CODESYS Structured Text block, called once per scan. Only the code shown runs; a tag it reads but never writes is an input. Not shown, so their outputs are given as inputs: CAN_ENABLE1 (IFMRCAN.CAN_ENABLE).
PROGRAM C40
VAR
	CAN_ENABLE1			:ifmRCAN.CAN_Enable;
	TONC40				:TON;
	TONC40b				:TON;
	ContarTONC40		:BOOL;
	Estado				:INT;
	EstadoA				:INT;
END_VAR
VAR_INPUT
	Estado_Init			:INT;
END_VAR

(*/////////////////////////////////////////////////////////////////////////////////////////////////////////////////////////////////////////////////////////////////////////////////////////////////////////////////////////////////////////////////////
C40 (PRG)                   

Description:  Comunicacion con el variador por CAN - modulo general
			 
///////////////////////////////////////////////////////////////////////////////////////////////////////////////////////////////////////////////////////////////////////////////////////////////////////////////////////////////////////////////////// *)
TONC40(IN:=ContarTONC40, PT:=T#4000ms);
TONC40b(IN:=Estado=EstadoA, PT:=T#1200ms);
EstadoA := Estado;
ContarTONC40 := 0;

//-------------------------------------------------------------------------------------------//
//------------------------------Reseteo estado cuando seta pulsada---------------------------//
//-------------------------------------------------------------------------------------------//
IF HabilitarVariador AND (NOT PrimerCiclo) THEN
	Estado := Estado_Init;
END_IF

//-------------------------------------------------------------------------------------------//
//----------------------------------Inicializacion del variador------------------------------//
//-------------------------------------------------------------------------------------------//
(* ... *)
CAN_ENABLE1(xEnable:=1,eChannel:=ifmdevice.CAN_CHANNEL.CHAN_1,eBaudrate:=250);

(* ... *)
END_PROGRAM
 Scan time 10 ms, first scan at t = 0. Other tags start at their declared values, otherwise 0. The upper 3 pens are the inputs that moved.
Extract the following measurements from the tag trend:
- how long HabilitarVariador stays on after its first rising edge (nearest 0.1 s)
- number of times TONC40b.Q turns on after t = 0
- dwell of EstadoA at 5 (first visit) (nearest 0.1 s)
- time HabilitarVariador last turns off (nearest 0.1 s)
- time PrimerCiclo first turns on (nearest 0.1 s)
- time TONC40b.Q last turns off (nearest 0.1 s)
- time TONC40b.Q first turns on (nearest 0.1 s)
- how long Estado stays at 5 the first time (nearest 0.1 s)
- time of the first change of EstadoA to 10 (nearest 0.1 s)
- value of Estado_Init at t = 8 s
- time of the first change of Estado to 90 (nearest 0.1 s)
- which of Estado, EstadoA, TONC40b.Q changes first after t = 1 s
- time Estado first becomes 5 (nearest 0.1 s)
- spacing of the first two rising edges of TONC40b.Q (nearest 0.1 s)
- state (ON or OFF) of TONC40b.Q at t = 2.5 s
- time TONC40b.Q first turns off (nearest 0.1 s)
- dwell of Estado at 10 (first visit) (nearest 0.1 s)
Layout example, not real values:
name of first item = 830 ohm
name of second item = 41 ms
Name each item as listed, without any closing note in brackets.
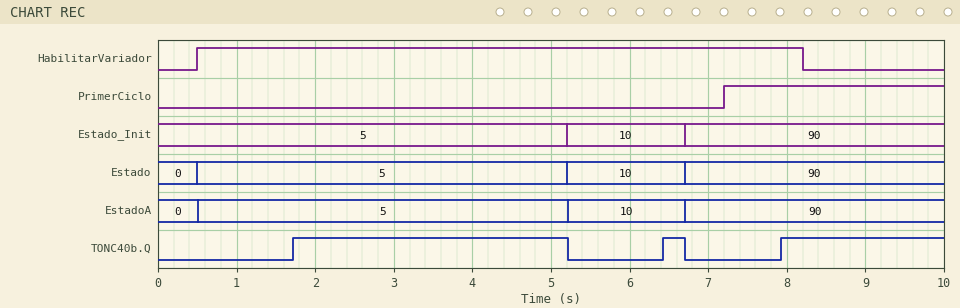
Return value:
how long HabilitarVariador stays on after its first rising edge = 7.7 s
number of times TONC40b.Q turns on after t = 0 = 3
dwell of EstadoA at 5 (first visit) = 4.7 s
time HabilitarVariador last turns off = 8.2 s
time PrimerCiclo first turns on = 7.2 s
time TONC40b.Q last turns off = 6.7 s
time TONC40b.Q first turns on = 1.7 s
how long Estado stays at 5 the first time = 4.7 s
time of the first change of EstadoA to 10 = 5.2 s
value of Estado_Init at t = 8 s = 90
time of the first change of Estado to 90 = 6.7 s
which of Estado, EstadoA, TONC40b.Q changes first after t = 1 s = TONC40b.Q
time Estado first becomes 5 = 0.5 s
spacing of the first two rising edges of TONC40b.Q = 4.7 s
state (ON or OFF) of TONC40b.Q at t = 2.5 s = ON
time TONC40b.Q first turns off = 5.2 s
dwell of Estado at 10 (first visit) = 1.5 s
